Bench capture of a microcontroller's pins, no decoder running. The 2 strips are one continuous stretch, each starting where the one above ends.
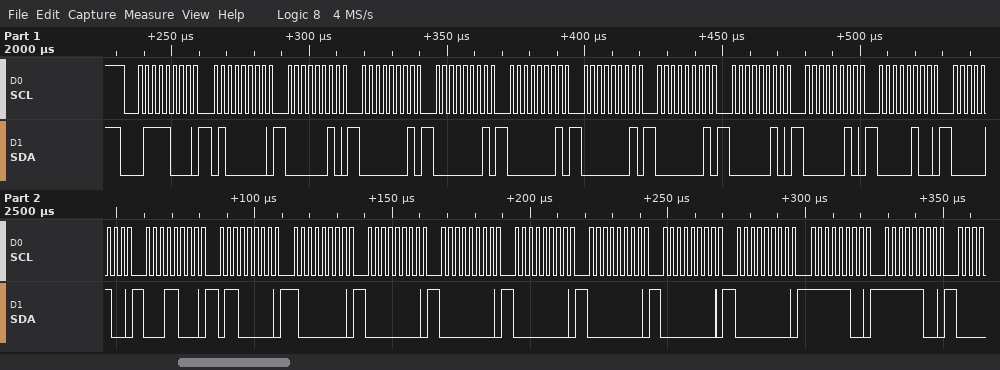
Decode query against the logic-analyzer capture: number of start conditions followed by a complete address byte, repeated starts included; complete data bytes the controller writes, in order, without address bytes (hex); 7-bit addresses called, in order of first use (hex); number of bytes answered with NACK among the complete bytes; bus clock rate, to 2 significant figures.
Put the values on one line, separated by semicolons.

1; 40 02 01 01 01 01 01 02 02 04 04 18 60 80 00 00 00 00 00 00 FC FC; 0x3C; 0; 400 kHz
